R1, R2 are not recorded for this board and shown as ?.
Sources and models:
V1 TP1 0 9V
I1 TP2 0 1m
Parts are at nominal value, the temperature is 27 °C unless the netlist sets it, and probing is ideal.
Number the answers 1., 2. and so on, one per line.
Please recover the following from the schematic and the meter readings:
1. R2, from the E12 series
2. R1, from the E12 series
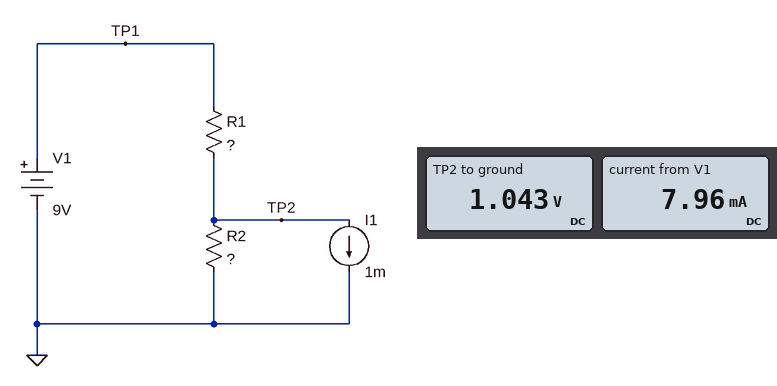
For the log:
1. 150 Ω
2. 1 kΩ
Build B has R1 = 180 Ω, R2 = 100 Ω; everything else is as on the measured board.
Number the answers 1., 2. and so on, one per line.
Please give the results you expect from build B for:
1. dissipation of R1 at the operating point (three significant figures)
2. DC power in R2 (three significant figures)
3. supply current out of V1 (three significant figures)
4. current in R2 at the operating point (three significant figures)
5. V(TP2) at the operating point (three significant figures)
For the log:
1. 190 mW
2. 99.2 mW
3. 32.5 mA
4. 31.5 mA
5. 3.15 V
